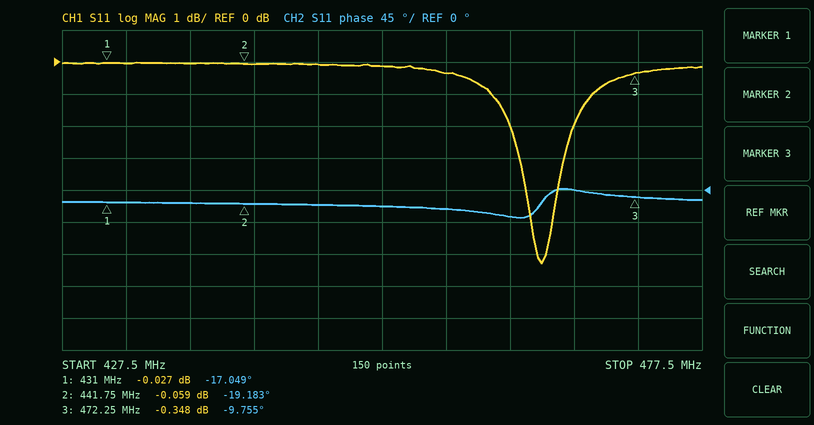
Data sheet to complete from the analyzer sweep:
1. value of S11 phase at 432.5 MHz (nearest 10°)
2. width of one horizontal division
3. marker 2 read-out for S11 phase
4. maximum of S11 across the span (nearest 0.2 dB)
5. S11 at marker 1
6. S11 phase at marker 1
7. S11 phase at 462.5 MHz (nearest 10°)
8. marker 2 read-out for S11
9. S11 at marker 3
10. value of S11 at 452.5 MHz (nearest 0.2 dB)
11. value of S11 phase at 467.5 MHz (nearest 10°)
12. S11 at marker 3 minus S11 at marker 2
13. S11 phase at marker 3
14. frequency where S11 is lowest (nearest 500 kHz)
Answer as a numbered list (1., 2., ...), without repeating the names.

1. -20°
2. 5 MHz
3. -19.183°
4. 0.0 dB
5. -0.027 dB
6. -17.049°
7. -40°
8. -0.059 dB
9. -0.348 dB
10. -0.2 dB
11. 0°
12. -0.289 dB
13. -9.755°
14. 465.0 MHz
